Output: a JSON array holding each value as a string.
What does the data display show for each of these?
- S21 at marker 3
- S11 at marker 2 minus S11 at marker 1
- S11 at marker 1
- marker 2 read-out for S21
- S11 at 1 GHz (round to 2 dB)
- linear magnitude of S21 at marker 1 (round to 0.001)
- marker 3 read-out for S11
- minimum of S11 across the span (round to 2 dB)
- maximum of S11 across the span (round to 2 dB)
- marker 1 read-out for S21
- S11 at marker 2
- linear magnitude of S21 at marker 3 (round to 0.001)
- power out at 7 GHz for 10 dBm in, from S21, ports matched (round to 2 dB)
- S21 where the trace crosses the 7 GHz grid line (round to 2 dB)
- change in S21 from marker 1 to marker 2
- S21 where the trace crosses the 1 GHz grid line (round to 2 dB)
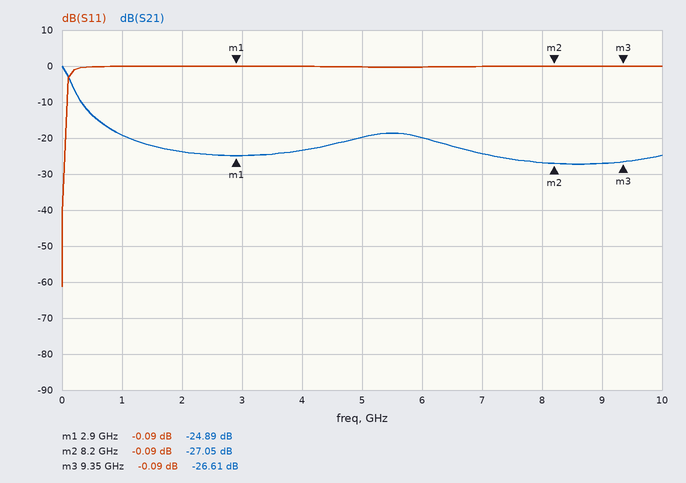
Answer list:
["-26.61 dB", "0.00 dB", "-0.09 dB", "-27.05 dB", "0 dB", "0.057", "-0.09 dB", "-62 dB", "0 dB", "-24.89 dB", "-0.09 dB", "0.047", "-14 dBm", "-24 dB", "-2.16 dB", "-20 dB"]
